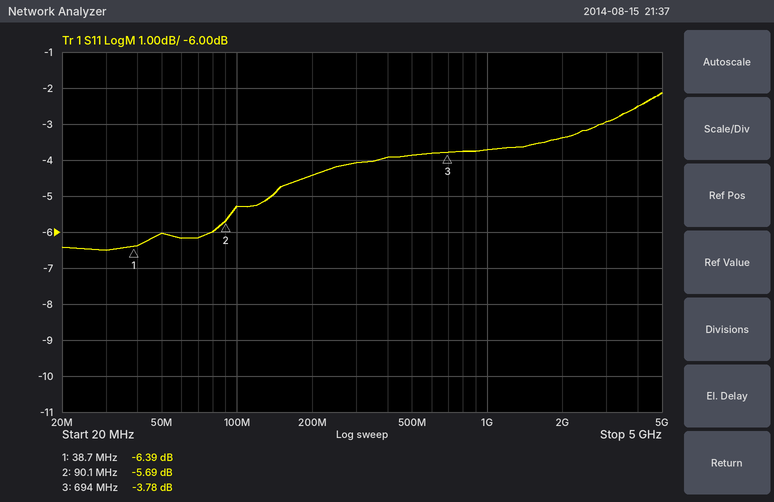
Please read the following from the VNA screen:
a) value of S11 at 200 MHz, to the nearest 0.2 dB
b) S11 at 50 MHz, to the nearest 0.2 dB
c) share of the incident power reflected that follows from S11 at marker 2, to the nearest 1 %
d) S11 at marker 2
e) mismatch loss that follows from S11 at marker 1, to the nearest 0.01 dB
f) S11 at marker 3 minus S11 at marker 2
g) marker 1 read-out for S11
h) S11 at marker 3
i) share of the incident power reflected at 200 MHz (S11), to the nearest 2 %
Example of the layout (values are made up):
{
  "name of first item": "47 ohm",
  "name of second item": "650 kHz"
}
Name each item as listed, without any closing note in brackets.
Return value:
{
  "value of S11 at 200 MHz, to the nearest 0.2 dB": "-4.4 dB",
  "S11 at 50 MHz, to the nearest 0.2 dB": "-6.0 dB",
  "share of the incident power reflected that follows from S11 at marker 2, to the nearest 1 %": "27 %",
  "S11 at marker 2": "-5.69 dB",
  "mismatch loss that follows from S11 at marker 1, to the nearest 0.01 dB": "1.13 dB",
  "S11 at marker 3 minus S11 at marker 2": "1.91 dB",
  "marker 1 read-out for S11": "-6.39 dB",
  "S11 at marker 3": "-3.78 dB",
  "share of the incident power reflected at 200 MHz (S11), to the nearest 2 %": "36 %"
}
